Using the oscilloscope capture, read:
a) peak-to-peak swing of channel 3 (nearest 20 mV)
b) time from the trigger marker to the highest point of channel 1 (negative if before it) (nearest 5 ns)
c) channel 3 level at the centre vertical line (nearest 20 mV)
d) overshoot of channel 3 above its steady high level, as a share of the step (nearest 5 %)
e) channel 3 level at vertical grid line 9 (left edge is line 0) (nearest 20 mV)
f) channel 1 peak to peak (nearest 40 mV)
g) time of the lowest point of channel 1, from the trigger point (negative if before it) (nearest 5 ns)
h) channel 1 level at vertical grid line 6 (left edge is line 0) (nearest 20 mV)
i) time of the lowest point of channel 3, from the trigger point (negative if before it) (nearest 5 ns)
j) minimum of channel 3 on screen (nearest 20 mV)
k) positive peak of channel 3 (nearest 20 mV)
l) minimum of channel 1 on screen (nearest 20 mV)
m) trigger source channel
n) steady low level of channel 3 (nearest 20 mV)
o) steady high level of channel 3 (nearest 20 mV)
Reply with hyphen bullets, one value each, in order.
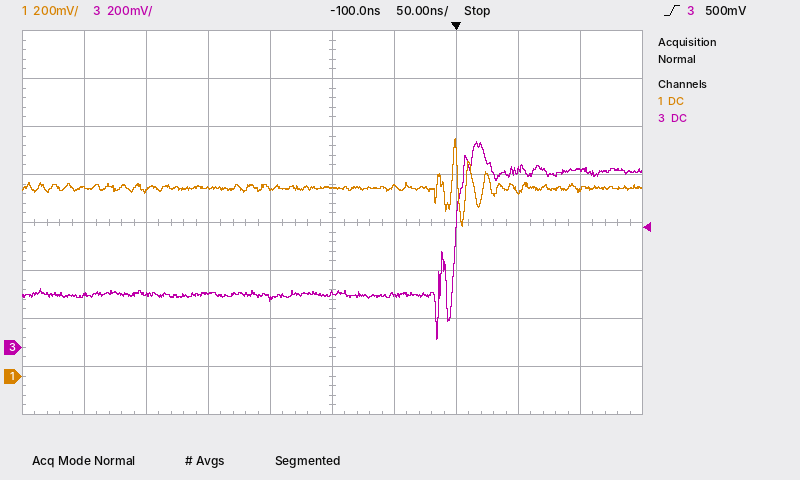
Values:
- 820 mV
- 0 ns
- 220 mV
- 25 %
- 740 mV
- 360 mV
- +5 ns
- 780 mV
- -15 ns
- 40 mV
- 860 mV
- 620 mV
- channel 3
- 220 mV
- 740 mV
